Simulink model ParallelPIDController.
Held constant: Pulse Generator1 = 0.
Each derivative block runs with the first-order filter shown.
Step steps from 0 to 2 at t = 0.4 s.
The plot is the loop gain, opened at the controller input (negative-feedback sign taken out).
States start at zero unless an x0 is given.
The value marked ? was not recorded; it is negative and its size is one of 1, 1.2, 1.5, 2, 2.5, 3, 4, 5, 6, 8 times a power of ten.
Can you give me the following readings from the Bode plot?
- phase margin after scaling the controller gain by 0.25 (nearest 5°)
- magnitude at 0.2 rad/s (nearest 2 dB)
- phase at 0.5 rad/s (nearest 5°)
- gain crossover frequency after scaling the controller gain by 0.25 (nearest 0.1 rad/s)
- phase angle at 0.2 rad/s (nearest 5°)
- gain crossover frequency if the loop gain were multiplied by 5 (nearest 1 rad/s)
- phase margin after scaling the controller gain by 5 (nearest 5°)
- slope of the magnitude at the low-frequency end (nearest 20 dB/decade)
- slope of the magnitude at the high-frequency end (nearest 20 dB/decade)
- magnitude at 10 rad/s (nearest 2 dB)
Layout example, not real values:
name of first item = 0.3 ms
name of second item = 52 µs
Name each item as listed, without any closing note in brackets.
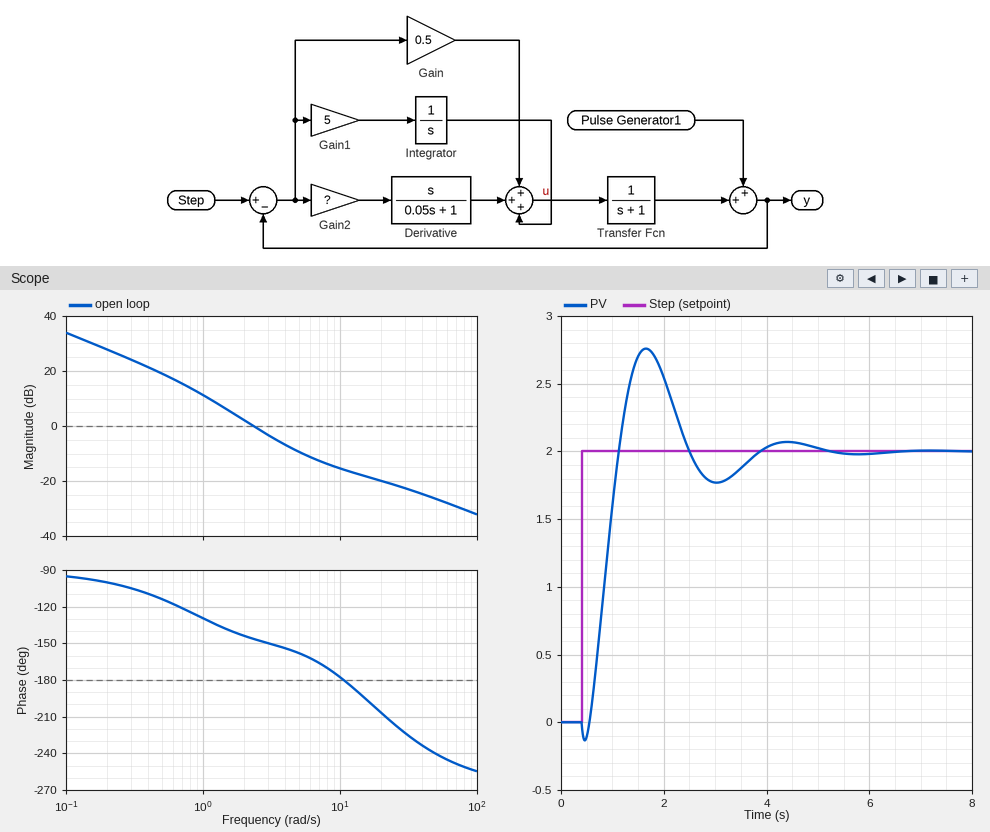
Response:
phase margin after scaling the controller gain by 0.25 = 50°
magnitude at 0.2 rad/s = 28 dB
phase at 0.5 rad/s = -115°
gain crossover frequency after scaling the controller gain by 0.25 = 0.9 rad/s
phase angle at 0.2 rad/s = -100°
gain crossover frequency if the loop gain were multiplied by 5 = 8 rad/s
phase margin after scaling the controller gain by 5 = 10°
slope of the magnitude at the low-frequency end = -20 dB/decade
slope of the magnitude at the high-frequency end = -20 dB/decade
magnitude at 10 rad/s = -16 dB
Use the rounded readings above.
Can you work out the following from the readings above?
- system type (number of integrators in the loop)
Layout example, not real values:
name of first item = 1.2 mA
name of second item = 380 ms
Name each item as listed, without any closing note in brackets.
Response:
system type = 1
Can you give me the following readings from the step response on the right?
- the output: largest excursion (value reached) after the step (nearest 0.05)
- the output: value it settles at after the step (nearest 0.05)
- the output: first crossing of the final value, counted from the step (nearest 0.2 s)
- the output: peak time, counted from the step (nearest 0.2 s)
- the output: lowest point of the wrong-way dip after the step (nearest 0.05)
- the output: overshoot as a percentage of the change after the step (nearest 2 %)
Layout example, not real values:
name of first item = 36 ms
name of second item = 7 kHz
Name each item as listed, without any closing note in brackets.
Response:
the output: largest excursion (value reached) after the step = 2.75
the output: value it settles at after the step = 2.00
the output: first crossing of the final value, counted from the step = 0.8 s
the output: peak time, counted from the step = 1.2 s
the output: lowest point of the wrong-way dip after the step = -0.15
the output: overshoot as a percentage of the change after the step = 38 %
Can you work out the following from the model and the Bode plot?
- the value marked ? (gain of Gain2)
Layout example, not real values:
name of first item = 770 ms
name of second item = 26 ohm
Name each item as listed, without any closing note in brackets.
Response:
the value marked ? = -0.15
